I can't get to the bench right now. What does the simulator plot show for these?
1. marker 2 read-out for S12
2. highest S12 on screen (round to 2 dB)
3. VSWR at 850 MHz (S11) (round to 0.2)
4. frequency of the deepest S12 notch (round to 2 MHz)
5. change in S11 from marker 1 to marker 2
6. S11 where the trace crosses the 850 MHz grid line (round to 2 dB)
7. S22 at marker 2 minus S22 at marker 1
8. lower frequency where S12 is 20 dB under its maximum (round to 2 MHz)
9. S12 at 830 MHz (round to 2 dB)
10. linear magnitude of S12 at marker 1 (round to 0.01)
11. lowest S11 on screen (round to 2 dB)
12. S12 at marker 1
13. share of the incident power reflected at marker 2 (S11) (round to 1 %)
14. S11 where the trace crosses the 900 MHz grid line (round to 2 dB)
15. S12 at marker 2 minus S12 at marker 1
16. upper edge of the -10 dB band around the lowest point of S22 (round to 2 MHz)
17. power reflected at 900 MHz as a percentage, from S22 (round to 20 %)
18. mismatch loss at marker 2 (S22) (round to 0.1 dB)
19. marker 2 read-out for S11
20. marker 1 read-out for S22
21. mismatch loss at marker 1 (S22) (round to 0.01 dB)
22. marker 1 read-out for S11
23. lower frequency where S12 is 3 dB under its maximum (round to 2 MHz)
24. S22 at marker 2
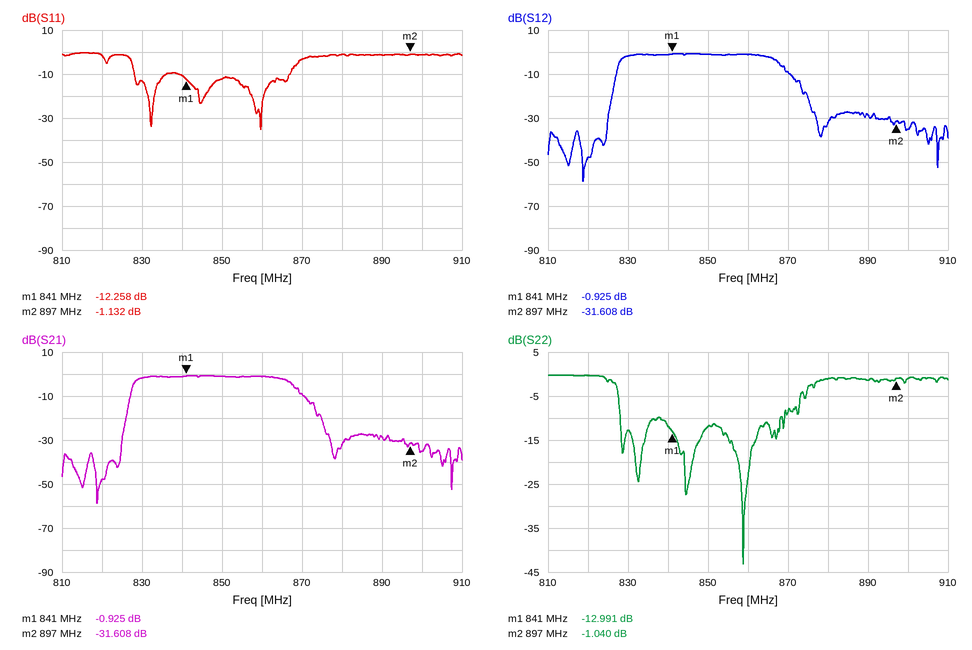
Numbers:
-31.608 dB
0 dB
1.6
818 MHz
11.126 dB
-12 dB
11.951 dB
826 MHz
-2 dB
0.90
-36 dB
-0.925 dB
77 %
-2 dB
-30.683 dB
868 MHz
80 %
6.7 dB
-1.132 dB
-12.991 dB
0.22 dB
-12.258 dB
828 MHz
-1.040 dB
